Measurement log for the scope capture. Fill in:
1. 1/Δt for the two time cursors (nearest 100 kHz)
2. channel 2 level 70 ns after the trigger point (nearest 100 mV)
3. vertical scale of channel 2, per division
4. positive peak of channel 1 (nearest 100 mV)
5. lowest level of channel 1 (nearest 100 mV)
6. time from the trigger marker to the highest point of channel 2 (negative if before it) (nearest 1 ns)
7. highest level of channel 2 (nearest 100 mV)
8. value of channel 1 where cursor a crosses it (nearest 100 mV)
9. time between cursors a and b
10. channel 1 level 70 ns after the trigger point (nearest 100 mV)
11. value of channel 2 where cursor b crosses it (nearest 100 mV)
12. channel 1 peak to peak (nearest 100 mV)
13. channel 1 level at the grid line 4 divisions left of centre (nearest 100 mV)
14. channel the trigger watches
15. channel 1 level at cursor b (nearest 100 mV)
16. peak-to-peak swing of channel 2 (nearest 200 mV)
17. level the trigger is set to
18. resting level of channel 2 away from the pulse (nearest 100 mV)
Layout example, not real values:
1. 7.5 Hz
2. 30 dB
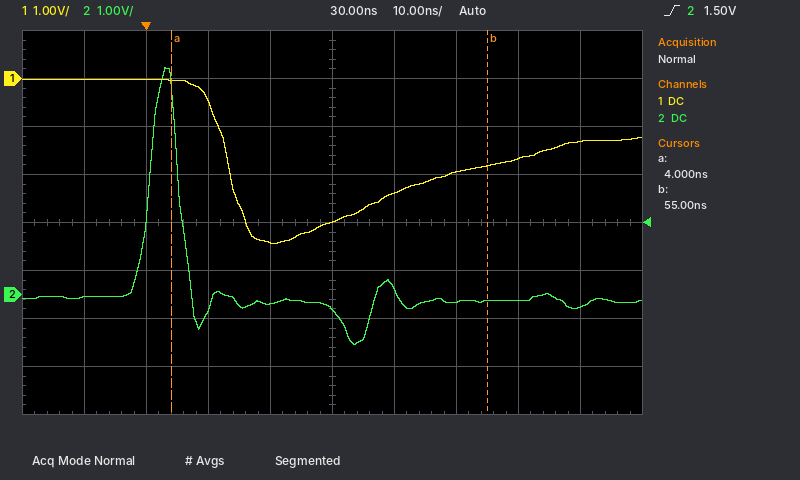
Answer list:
1. 19.6 MHz
2. -300 mV
3. 1 V
4. 0.0 V
5. -3.4 V
6. +3 ns
7. 4.7 V
8. 0.0 V
9. 51 ns
10. -1.3 V
11. -100 mV
12. 3.4 V
13. 0.0 V
14. channel 2
15. -1.8 V
16. 5.8 V
17. 1.50 V
18. -100 mV
